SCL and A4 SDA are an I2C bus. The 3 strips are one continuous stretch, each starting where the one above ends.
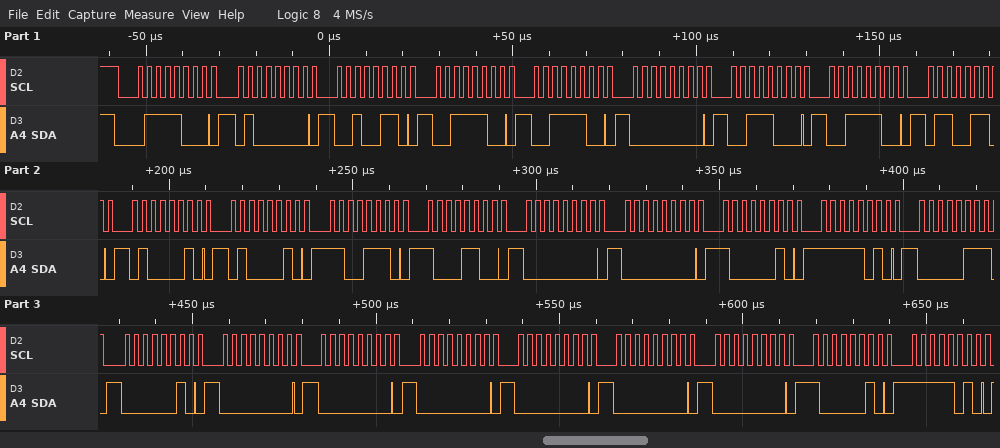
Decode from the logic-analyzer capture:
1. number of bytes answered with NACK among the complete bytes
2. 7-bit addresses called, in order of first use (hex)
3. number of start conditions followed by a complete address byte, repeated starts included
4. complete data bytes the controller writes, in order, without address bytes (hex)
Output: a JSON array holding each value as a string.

["0", "0x3C", "1", "40 26 3C 3C 00 38 3C 66 42 42 CE 8C 00 00 82 FA 07 02 00 00 00 00 00 00 82 FA"]
